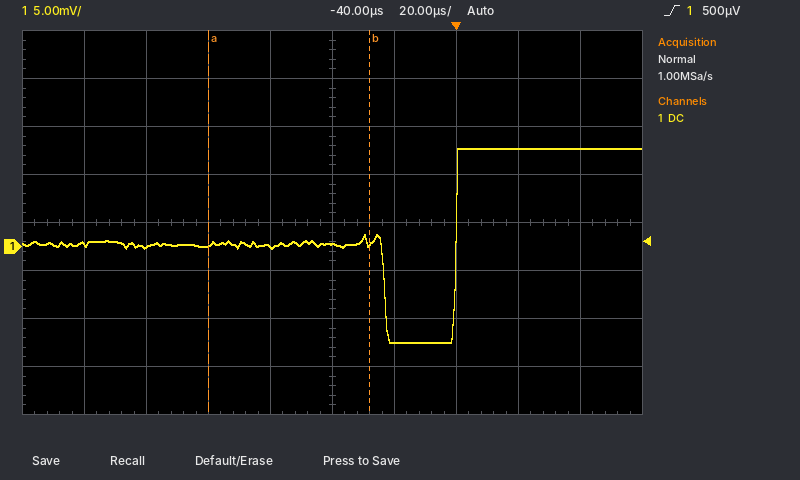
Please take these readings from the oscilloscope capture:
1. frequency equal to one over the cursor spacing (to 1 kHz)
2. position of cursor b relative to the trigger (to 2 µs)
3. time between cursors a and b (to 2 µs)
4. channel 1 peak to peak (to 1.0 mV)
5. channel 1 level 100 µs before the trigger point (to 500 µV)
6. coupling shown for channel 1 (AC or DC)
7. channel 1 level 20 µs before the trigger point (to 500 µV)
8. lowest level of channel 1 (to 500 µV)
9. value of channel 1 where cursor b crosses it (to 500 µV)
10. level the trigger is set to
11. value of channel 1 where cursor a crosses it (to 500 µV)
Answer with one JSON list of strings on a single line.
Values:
["19 kHz", "-28 µs", "52 µs", "20.0 mV", "0.0 mV", "DC", "-10.0 mV", "-10.0 mV", "500 µV", "500 µV", "0.0 mV"]
